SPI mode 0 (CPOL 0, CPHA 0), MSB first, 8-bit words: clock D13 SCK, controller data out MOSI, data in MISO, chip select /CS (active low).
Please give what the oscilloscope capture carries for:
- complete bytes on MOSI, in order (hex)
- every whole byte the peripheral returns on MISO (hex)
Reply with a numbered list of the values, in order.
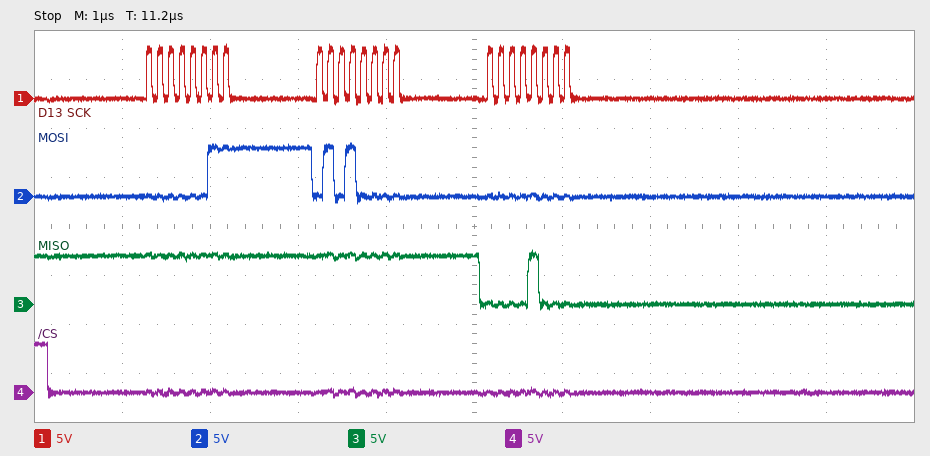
1. 03 50 00
2. FF FF 08
